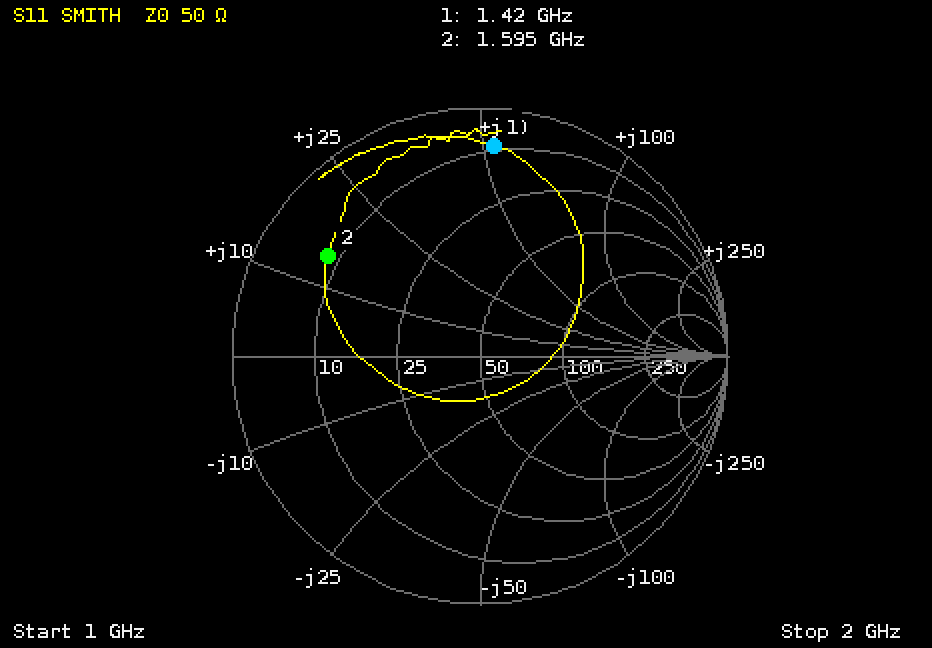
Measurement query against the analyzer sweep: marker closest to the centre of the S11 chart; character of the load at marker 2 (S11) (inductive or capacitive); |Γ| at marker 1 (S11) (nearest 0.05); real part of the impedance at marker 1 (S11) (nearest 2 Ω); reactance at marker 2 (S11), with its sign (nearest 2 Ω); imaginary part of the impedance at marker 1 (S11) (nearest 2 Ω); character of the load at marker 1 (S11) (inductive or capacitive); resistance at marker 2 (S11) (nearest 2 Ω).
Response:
marker 2
inductive
0.85
8 Ω
+14 Ω
+52 Ω
inductive
8 Ω
